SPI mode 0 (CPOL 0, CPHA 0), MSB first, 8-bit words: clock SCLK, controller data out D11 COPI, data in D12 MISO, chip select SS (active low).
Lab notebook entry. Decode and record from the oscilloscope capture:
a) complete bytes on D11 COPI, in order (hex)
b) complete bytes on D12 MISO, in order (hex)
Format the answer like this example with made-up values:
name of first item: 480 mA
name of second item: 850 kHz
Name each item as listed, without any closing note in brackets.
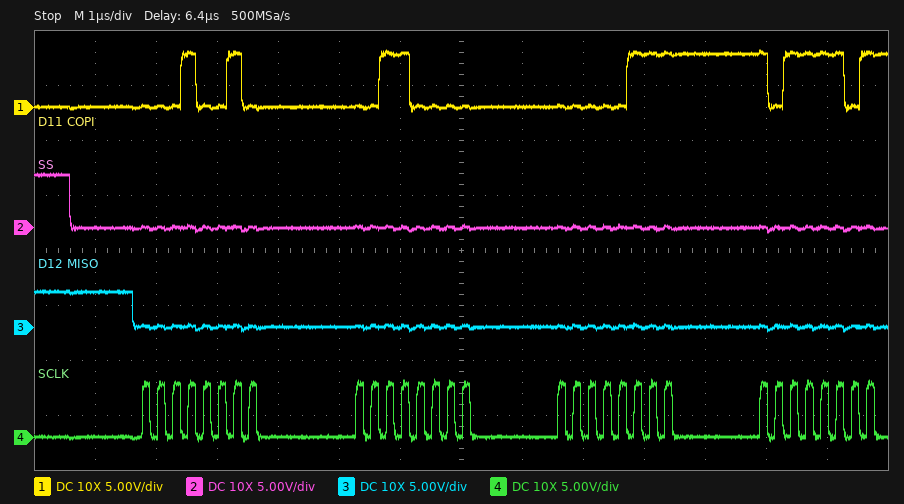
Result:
complete bytes on D11 COPI, in order: 12 30 07 BD
complete bytes on D12 MISO, in order: 00 00 00 00
